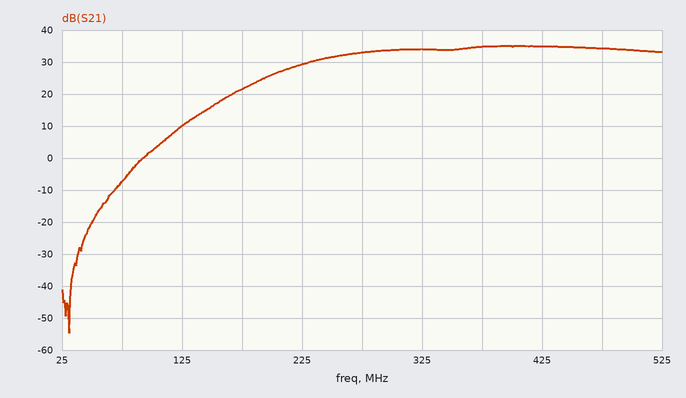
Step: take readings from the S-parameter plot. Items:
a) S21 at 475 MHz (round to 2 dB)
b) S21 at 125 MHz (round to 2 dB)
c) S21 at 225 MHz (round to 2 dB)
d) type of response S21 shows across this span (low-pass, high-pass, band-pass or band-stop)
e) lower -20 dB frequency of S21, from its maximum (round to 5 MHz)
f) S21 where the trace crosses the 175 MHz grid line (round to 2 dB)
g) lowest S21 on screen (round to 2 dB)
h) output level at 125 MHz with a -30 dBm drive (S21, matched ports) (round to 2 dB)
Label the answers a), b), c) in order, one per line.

a) 34 dB
b) 10 dB
c) 30 dB
d) high-pass
e) 145 MHz
f) 22 dB
g) -54 dB
h) -20 dBm
